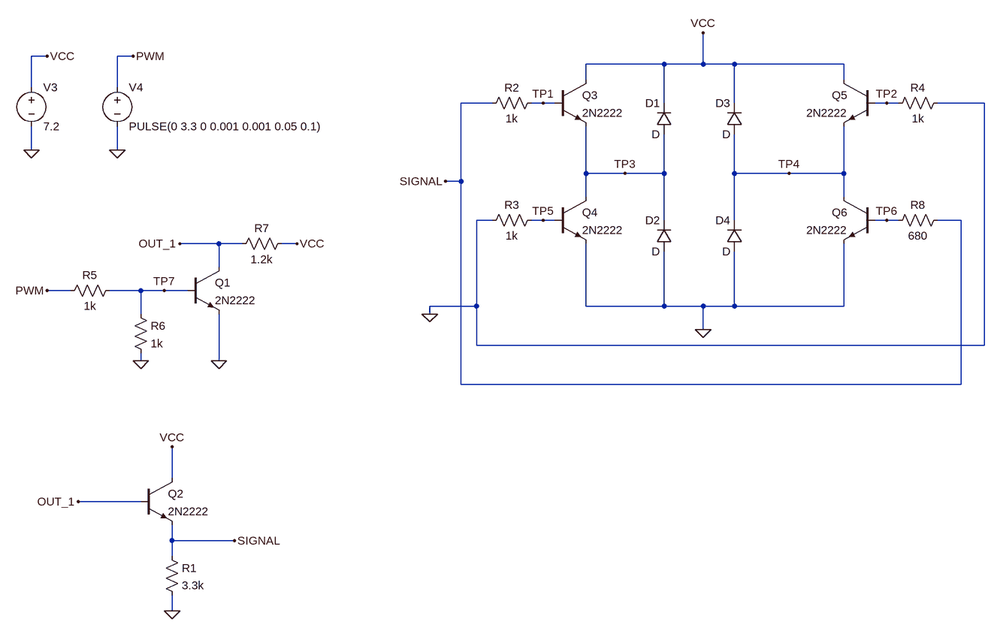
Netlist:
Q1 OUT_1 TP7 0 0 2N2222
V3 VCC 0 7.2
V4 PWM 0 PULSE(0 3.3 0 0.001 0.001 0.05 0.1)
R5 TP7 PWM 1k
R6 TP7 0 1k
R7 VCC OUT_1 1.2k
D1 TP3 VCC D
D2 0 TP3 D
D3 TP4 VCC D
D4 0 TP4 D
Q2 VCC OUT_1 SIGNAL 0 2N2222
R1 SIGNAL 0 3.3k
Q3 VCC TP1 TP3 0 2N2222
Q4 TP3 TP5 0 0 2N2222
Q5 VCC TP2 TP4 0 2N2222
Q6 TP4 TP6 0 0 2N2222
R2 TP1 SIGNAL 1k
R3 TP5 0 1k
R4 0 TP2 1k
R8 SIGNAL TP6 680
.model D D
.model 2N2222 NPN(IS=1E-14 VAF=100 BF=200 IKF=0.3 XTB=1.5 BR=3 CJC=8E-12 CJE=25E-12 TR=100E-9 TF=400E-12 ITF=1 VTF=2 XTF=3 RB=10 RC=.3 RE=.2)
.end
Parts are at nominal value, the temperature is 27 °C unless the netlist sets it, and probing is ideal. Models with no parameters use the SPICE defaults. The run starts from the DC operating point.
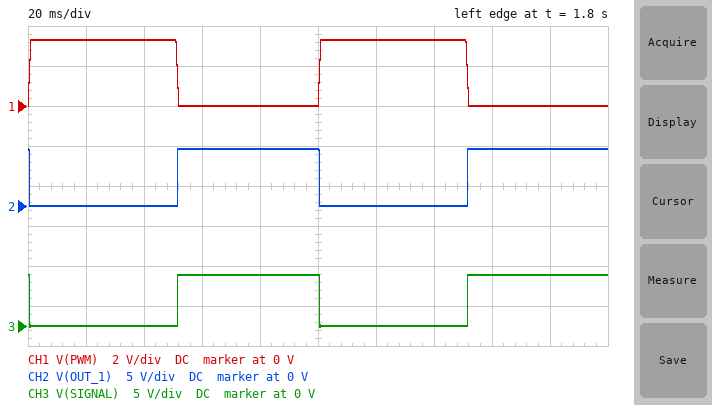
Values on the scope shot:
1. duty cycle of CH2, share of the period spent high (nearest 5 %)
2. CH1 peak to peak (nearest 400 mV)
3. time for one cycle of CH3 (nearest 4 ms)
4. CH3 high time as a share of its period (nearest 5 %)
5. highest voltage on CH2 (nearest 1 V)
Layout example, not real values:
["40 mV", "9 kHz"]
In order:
["50 %", "3.2 V", "100 ms", "50 %", "7 V"]
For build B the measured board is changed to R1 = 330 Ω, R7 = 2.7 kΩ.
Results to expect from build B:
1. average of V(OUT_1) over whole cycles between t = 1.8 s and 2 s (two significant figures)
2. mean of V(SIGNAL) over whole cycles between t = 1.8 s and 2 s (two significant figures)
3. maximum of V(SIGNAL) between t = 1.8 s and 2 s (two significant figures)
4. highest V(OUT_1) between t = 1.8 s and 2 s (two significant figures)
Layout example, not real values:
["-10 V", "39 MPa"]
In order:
["3.3 V", "3.0 V", "6.1 V", "6.8 V"]
